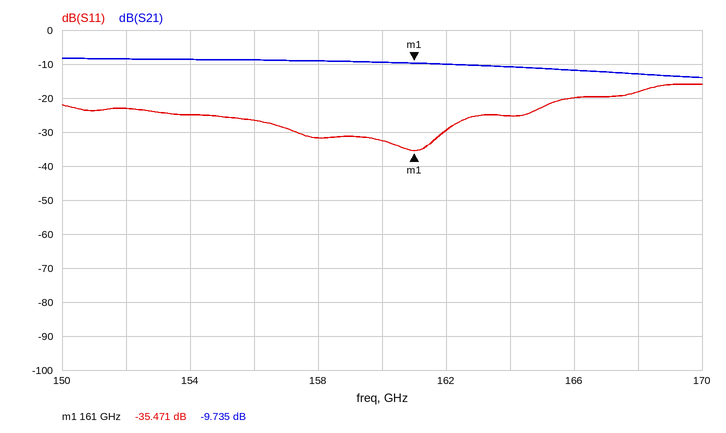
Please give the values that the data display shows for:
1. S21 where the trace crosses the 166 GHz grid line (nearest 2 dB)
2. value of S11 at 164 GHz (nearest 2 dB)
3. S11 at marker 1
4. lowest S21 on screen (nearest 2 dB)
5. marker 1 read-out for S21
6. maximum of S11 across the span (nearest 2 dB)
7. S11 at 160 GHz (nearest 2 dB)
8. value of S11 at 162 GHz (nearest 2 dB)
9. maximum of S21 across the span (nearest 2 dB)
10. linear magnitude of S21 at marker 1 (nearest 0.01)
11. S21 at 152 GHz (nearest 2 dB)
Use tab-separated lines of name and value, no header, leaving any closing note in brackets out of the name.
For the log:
S21 where the trace crosses the 166 GHz grid line	-12 dB
value of S11 at 164 GHz	-26 dB
S11 at marker 1	-35.471 dB
lowest S21 on screen	-14 dB
marker 1 read-out for S21	-9.735 dB
maximum of S11 across the span	-16 dB
S11 at 160 GHz	-32 dB
value of S11 at 162 GHz	-30 dB
maximum of S21 across the span	-8 dB
linear magnitude of S21 at marker 1	0.33
S21 at 152 GHz	-8 dB
